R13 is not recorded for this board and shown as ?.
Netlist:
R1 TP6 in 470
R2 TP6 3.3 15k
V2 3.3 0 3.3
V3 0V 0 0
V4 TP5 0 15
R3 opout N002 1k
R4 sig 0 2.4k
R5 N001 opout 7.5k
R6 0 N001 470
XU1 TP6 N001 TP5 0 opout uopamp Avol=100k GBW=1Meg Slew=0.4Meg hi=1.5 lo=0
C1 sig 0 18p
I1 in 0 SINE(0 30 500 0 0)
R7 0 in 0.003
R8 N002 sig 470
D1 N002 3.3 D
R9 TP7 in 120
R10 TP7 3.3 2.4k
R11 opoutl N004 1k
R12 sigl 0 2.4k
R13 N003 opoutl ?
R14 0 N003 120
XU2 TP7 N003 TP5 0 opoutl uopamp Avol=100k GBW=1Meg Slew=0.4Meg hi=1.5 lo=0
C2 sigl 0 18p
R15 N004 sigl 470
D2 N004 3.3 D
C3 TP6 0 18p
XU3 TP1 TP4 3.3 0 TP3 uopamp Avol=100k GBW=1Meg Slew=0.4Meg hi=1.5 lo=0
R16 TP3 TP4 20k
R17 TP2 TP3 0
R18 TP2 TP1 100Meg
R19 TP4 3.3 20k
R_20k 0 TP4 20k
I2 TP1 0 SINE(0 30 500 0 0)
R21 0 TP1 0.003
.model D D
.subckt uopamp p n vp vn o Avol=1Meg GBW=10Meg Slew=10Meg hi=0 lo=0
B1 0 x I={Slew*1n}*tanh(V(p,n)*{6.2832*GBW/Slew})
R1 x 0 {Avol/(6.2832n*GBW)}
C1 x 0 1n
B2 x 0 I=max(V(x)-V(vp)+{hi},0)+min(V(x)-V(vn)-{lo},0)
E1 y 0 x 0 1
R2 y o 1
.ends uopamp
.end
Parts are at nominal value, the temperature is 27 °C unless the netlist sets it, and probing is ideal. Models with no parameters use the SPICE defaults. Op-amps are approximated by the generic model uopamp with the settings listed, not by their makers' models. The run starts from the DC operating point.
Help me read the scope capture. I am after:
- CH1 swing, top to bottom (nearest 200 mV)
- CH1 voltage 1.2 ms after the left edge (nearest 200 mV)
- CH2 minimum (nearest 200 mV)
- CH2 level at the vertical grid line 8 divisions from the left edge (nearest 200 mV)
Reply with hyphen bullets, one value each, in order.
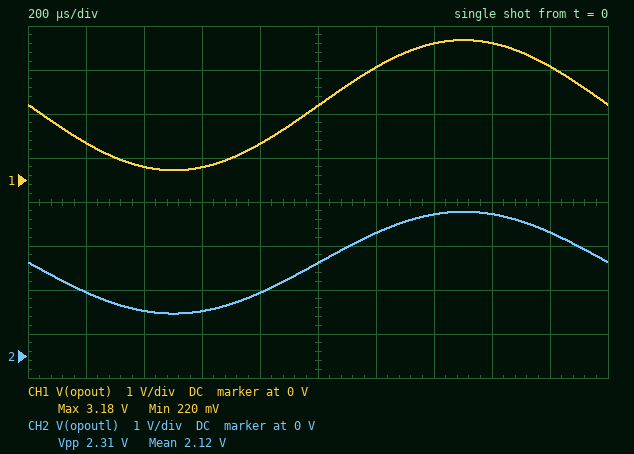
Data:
- 3.0 V
- 2.6 V
- 1.0 V
- 3.2 V
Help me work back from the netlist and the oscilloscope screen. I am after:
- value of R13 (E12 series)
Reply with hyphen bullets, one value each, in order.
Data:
- 1.5 kΩ
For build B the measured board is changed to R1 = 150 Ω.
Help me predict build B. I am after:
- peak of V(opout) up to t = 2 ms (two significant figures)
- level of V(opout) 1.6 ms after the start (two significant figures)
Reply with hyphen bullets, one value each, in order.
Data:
- 2.1 V
- 2.0 V
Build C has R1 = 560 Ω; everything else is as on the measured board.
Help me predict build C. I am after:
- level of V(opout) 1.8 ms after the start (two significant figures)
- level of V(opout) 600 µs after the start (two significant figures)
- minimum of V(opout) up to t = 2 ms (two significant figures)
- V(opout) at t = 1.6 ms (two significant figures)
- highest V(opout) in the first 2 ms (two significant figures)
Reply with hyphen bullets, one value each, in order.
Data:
- 2.9 V
- 610 mV
- 540 mV
- 3.4 V
- 3.5 V
